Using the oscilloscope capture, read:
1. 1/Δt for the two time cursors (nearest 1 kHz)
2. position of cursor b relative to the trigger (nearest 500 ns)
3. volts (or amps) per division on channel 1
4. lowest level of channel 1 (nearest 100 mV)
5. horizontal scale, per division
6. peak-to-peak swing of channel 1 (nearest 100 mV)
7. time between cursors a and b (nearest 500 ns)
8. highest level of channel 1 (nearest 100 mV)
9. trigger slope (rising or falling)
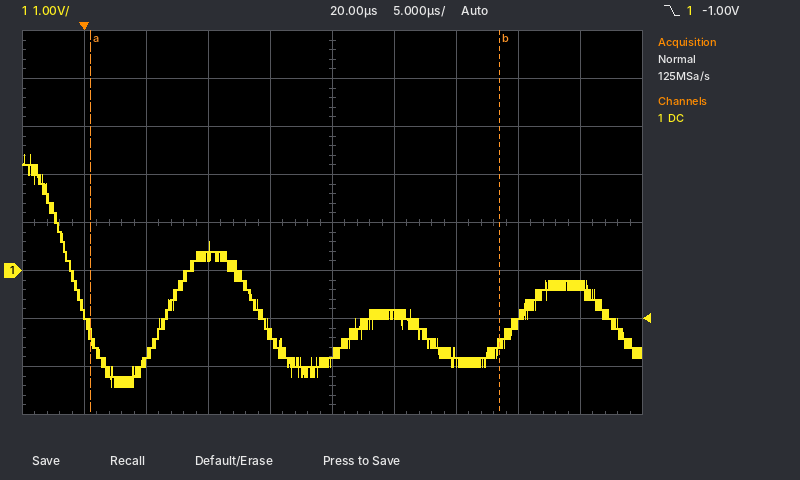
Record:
30 kHz
+33.5 µs
1 V
-2.4 V
5 µs
4.8 V
33.0 µs
2.4 V
falling
